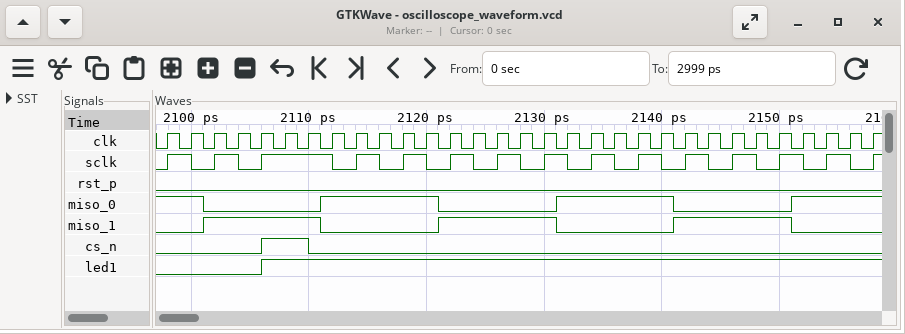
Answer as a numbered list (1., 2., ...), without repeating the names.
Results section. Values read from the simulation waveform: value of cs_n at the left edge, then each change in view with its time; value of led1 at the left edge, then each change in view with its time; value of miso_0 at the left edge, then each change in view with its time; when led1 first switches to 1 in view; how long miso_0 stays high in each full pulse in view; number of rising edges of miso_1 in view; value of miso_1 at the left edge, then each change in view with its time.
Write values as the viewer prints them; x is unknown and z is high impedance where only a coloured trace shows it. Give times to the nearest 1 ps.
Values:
1. 0, 1 at 2106 ps, 0 at 2110 ps
2. 0, 1 at 2106 ps
3. 1, 0 at 2101 ps, 1 at 2111 ps, 0 at 2121 ps, 1 at 2131 ps, 0 at 2141 ps, 1 at 2151 ps
4. 2106 ps
5. 10 ps, 10 ps
6. 3
7. 0, 1 at 2101 ps, 0 at 2111 ps, 1 at 2121 ps, 0 at 2131 ps, 1 at 2141 ps, 0 at 2151 ps
